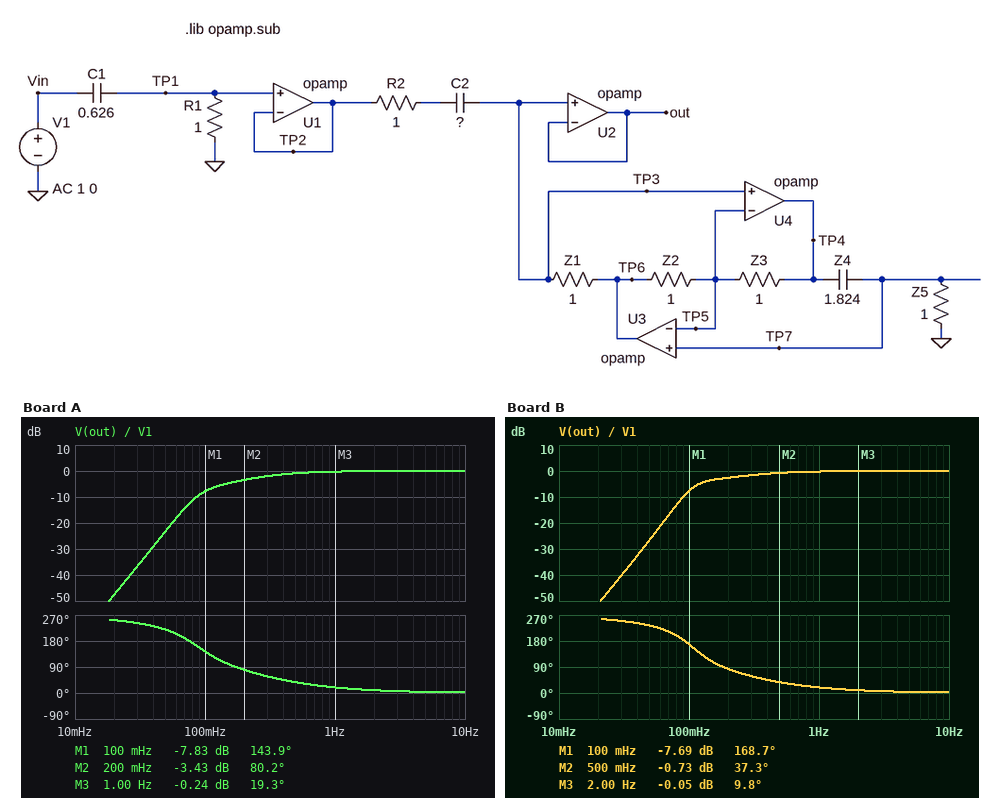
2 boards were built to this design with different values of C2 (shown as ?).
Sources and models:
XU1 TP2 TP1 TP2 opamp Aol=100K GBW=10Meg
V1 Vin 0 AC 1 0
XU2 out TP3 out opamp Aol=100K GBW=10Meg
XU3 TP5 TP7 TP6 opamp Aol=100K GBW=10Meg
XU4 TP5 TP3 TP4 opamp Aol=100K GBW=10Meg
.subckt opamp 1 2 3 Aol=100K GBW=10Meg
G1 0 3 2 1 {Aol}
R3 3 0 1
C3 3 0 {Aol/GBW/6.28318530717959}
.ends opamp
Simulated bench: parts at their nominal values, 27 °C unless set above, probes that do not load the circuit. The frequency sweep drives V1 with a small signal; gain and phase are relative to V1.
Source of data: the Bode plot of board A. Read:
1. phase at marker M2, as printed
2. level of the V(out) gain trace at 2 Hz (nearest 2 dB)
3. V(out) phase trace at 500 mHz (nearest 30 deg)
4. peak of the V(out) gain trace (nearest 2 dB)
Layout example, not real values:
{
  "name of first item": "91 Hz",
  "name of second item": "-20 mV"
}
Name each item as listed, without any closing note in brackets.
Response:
{
  "phase at marker M2, as printed": "80.2 deg",
  "level of the V(out) gain trace at 2 Hz": "0 dB",
  "V(out) phase trace at 500 mHz": "30 deg",
  "peak of the V(out) gain trace": "0 dB"
}
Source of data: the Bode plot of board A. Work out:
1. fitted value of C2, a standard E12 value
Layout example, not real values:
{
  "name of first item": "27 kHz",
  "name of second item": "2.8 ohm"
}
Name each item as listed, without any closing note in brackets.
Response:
{
  "fitted value of C2, a standard E12 value": "1.8 F"
}
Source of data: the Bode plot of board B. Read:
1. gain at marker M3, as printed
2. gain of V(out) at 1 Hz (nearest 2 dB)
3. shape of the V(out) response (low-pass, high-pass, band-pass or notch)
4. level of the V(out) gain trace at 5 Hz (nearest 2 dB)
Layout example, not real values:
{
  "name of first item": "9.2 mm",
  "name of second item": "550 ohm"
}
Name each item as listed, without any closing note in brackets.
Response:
{
  "gain at marker M3, as printed": "-0.05 dB",
  "gain of V(out) at 1 Hz": "0 dB",
  "shape of the V(out) response": "high-pass",
  "level of the V(out) gain trace at 5 Hz": "0 dB"
}
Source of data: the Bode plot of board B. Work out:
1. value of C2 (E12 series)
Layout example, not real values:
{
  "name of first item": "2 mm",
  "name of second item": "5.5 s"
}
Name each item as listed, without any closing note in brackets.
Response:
{
  "value of C2": "1.2 F"
}
